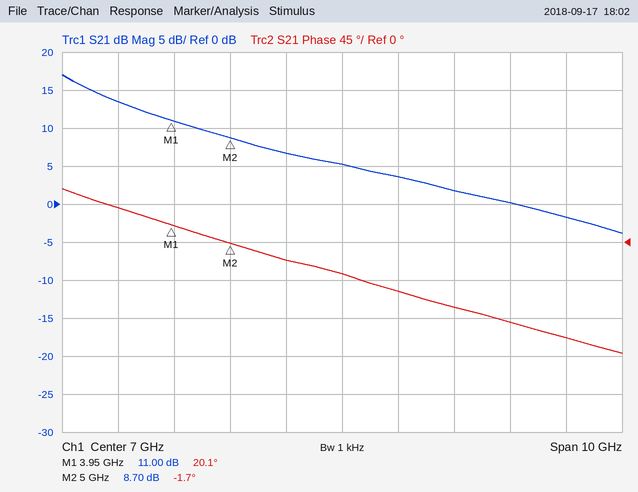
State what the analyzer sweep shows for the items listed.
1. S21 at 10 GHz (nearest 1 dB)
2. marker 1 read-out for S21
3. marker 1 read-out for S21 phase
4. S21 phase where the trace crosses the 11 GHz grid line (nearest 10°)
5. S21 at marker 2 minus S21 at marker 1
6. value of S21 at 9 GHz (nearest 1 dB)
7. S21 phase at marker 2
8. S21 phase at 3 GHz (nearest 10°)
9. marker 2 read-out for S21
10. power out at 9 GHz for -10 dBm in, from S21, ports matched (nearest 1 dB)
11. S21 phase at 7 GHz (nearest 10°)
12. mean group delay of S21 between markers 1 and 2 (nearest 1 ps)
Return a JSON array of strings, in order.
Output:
["0 dB", "11.00 dB", "20.1°", "-110°", "-2.30 dB", "2 dB", "-1.7°", "40°", "8.70 dB", "-8 dBm", "-40°", "58 ps"]
